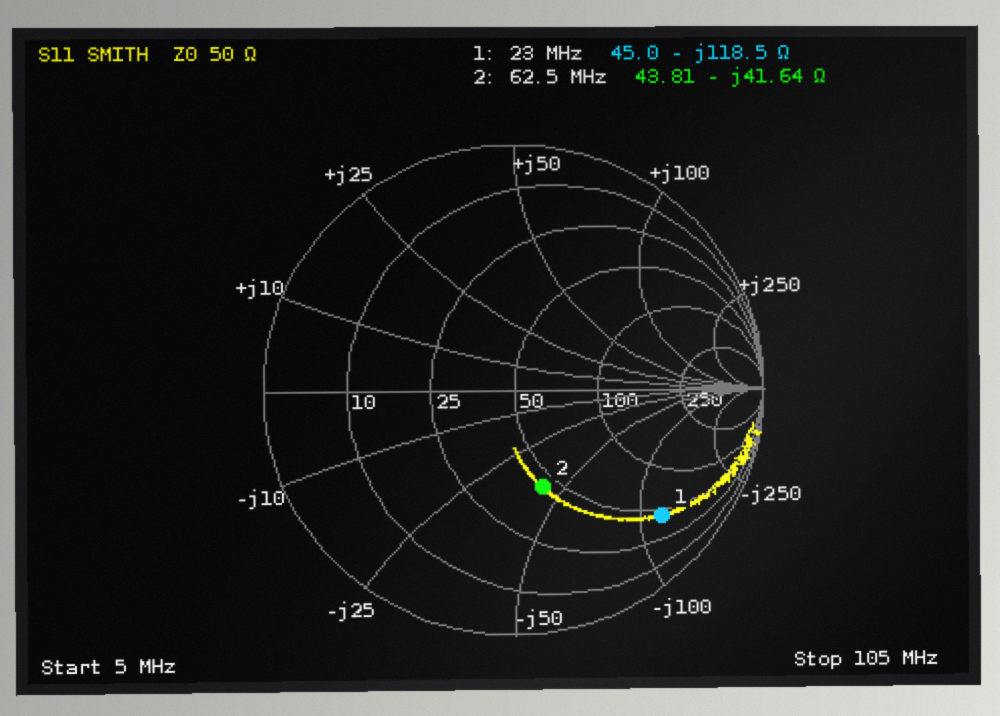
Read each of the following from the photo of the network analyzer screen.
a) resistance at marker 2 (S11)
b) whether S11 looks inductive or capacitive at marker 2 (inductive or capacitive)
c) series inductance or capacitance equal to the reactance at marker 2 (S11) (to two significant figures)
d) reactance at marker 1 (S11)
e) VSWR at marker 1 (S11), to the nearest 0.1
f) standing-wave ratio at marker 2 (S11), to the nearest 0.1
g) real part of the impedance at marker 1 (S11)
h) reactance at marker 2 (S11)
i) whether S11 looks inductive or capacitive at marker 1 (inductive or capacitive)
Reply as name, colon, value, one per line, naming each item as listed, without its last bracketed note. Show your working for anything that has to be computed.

resistance at marker 2: 43.81 Ω
whether S11 looks inductive or capacitive at marker 2: capacitive
series inductance or capacitance equal to the reactance at marker 2 (S11): C = 1/(2π × 62.5 MHz × 41.64 Ω) ≈ 61 pF
reactance at marker 1: -118.5 Ω
VSWR at marker 1 (S11), to the nearest 0.1: 8.1
standing-wave ratio at marker 2 (S11), to the nearest 0.1: 2.4
real part of the impedance at marker 1: 45.0 Ω
reactance at marker 2: -41.64 Ω
whether S11 looks inductive or capacitive at marker 1: capacitive
